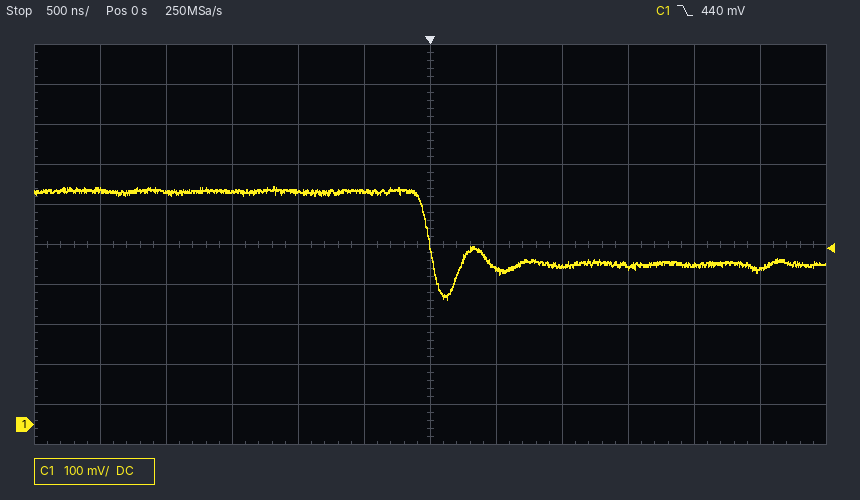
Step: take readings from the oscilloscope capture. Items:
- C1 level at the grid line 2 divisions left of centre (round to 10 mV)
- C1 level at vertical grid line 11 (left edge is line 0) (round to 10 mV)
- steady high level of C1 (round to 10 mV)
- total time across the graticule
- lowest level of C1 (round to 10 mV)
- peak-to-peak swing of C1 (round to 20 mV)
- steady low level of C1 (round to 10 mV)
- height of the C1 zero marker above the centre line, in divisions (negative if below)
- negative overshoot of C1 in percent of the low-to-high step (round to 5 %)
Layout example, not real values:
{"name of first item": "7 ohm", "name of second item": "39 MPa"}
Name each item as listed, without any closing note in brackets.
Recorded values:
{"C1 level at the grid line 2 divisions left of centre": "580 mV", "C1 level at vertical grid line 11 (left edge is line 0)": "390 mV", "steady high level of C1": "580 mV", "total time across the graticule": "6 µs", "lowest level of C1": "310 mV", "peak-to-peak swing of C1": "280 mV", "steady low level of C1": "400 mV", "height of the C1 zero marker above the centre line, in divisions": "-4.5 div", "negative overshoot of C1 in percent of the low-to-high step": "50 %"}
